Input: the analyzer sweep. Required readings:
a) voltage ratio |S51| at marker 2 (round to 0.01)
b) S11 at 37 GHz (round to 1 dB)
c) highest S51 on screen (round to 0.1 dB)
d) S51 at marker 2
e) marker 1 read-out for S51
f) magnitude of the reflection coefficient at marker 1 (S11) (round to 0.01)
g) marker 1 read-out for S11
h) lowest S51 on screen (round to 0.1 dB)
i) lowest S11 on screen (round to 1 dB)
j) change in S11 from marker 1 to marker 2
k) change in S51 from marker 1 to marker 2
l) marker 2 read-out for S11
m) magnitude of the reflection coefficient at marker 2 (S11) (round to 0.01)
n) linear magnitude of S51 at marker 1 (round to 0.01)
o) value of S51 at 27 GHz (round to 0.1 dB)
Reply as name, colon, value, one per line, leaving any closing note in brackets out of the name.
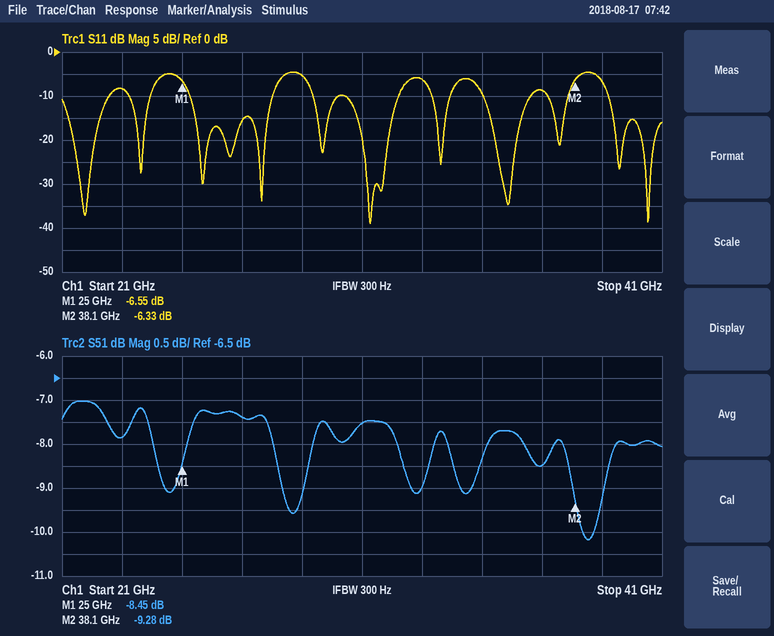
voltage ratio |S51| at marker 2: 0.34
S11 at 37 GHz: -9 dB
highest S51 on screen: -7.0 dB
S51 at marker 2: -9.28 dB
marker 1 read-out for S51: -8.45 dB
magnitude of the reflection coefficient at marker 1 (S11): 0.47
marker 1 read-out for S11: -6.55 dB
lowest S51 on screen: -10.2 dB
lowest S11 on screen: -39 dB
change in S11 from marker 1 to marker 2: 0.22 dB
change in S51 from marker 1 to marker 2: -0.83 dB
marker 2 read-out for S11: -6.33 dB
magnitude of the reflection coefficient at marker 2 (S11): 0.48
linear magnitude of S51 at marker 1: 0.38
value of S51 at 27 GHz: -7.4 dB
